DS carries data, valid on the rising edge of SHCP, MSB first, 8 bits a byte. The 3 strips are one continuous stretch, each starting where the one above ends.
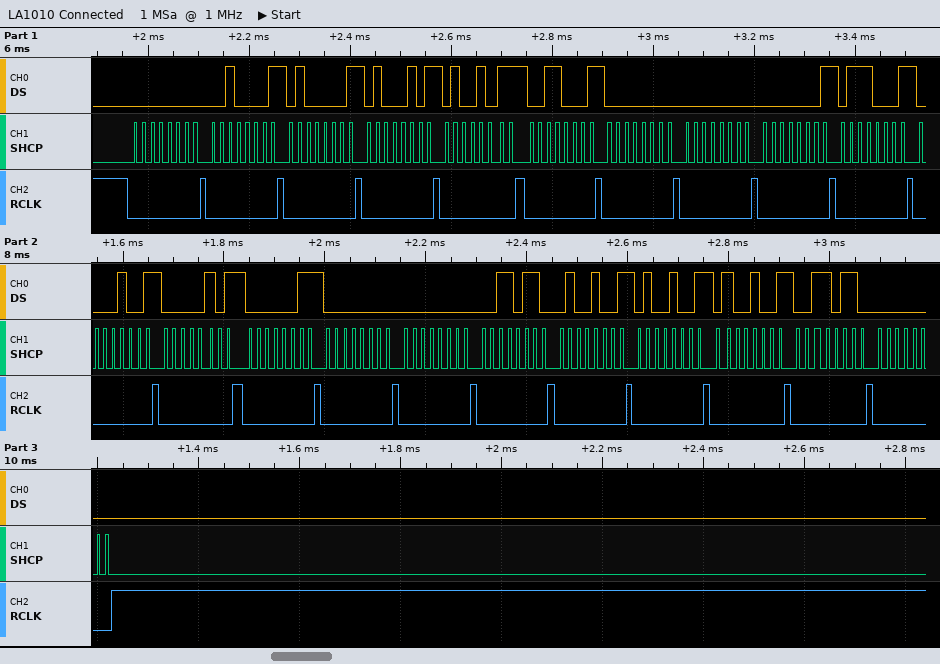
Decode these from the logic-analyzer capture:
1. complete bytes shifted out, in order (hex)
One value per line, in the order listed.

00 21 41 45 4B 31 00 00 01 71 09 05 03 00 00 36 49 49 49 36 00
